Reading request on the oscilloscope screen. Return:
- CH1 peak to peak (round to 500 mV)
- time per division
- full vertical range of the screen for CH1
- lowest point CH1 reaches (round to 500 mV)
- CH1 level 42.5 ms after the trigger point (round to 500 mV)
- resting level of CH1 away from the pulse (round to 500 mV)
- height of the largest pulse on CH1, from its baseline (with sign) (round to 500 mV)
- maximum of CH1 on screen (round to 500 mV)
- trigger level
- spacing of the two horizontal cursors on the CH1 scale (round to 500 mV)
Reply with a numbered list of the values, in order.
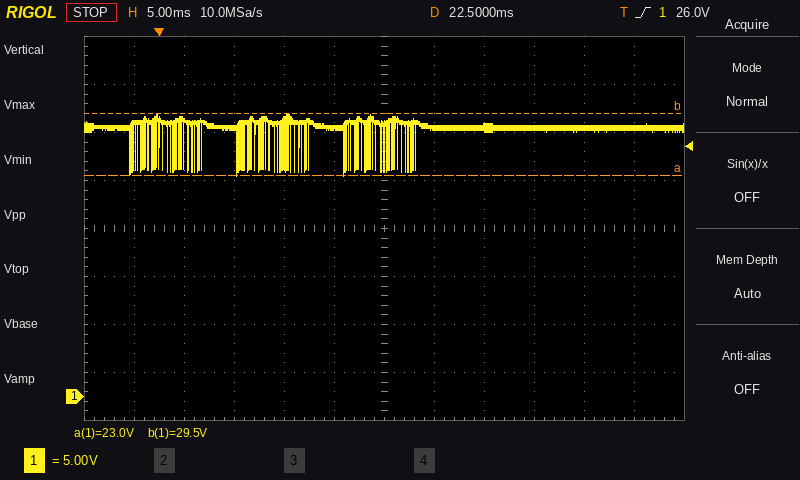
1. 6.5 V
2. 5 ms
3. 40 V
4. 23.0 V
5. 28.0 V
6. 28.0 V
7. -5.0 V
8. 29.5 V
9. 26.0 V
10. 6.5 V
